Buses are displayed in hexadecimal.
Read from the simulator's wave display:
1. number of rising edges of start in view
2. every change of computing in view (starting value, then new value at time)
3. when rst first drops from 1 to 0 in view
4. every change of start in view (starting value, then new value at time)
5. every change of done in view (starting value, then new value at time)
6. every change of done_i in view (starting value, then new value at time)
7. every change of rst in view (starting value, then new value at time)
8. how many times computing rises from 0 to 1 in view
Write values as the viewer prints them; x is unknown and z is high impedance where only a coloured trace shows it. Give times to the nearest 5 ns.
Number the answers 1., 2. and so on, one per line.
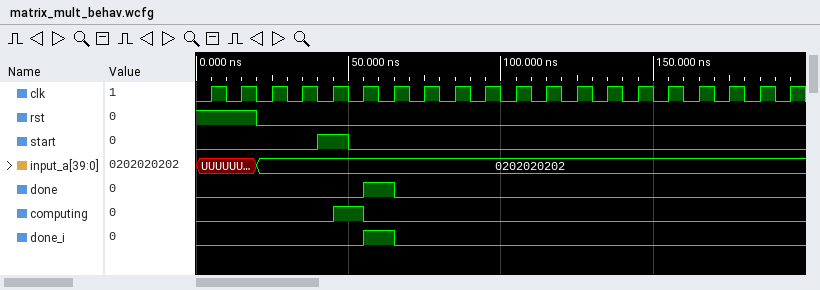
1. 1
2. 0, 1 at 45 ns, 0 at 55 ns
3. 20 ns
4. 0, 1 at 40 ns, 0 at 50 ns
5. 0, 1 at 55 ns, 0 at 65 ns
6. 0, 1 at 55 ns, 0 at 65 ns
7. 1, 0 at 20 ns
8. 1
